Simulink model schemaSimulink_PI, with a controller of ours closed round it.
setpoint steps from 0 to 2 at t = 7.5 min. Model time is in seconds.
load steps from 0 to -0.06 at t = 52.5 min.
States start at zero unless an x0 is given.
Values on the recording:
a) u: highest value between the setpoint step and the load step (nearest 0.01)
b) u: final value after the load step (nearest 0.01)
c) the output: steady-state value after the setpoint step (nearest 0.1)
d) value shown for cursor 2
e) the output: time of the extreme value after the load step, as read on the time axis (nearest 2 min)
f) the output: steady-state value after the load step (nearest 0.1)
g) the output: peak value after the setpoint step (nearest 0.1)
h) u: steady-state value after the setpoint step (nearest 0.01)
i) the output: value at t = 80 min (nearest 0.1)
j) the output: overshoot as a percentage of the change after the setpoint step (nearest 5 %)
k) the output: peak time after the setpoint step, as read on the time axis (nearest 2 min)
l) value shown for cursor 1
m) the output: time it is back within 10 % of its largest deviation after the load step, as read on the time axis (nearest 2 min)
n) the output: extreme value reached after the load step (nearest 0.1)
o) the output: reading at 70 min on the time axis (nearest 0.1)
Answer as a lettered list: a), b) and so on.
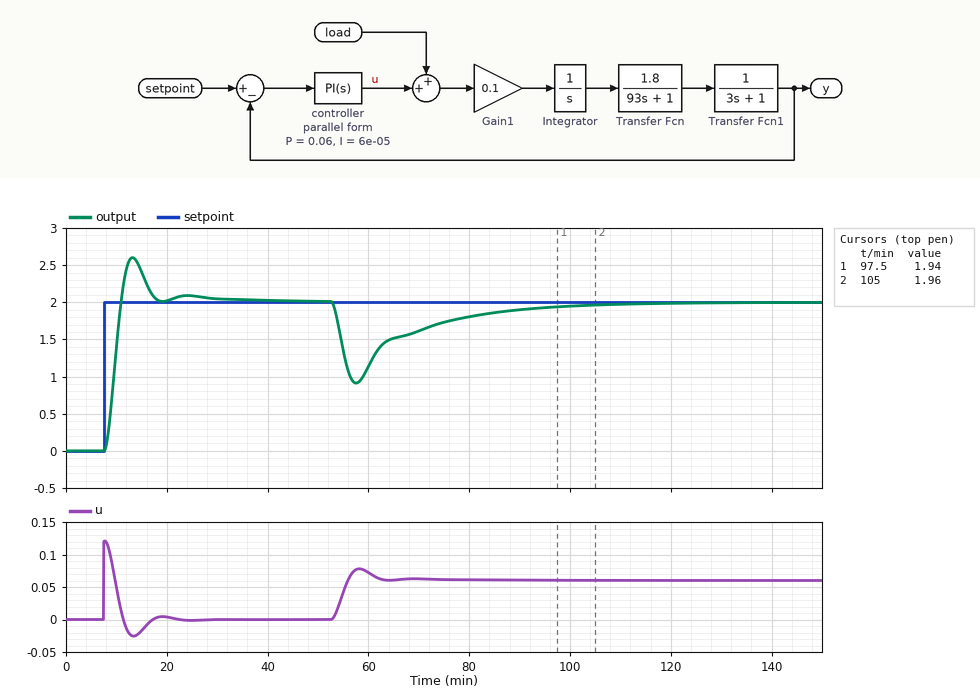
a) 0.12
b) 0.06
c) 2.0
d) 1.96
e) 58 min
f) 2.0
g) 2.6
h) 0.00
i) 1.8
j) 30 %
k) 14 min
l) 1.94
m) 88 min
n) 0.9
o) 1.6
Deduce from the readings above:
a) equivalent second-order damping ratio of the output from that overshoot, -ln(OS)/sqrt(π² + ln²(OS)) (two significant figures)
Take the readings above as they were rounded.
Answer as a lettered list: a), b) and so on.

a) 0.36
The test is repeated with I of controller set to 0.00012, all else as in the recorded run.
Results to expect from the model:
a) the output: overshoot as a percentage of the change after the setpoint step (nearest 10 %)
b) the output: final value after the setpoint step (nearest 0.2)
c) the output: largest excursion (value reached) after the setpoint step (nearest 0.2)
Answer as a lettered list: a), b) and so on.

a) 40 %
b) 2.0
c) 2.8
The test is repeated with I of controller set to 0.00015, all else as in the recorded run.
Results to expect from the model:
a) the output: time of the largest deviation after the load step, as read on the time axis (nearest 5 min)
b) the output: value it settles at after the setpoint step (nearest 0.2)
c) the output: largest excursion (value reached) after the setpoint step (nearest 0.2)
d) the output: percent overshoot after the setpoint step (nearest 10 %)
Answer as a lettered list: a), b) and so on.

a) 55 min
b) 2.0
c) 3.0
d) 50 %
